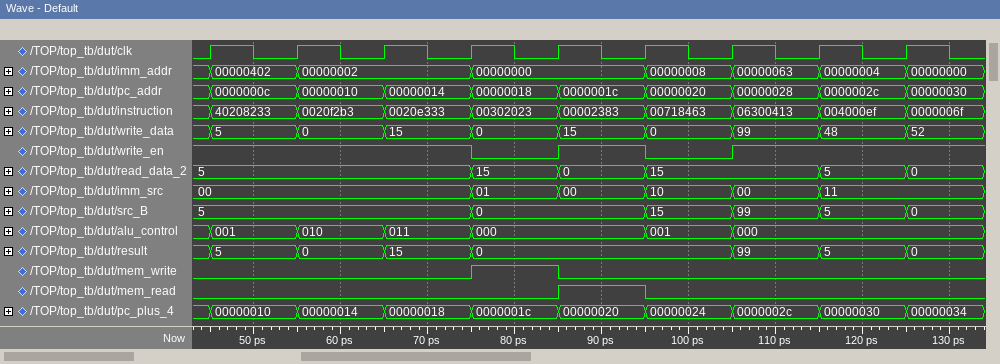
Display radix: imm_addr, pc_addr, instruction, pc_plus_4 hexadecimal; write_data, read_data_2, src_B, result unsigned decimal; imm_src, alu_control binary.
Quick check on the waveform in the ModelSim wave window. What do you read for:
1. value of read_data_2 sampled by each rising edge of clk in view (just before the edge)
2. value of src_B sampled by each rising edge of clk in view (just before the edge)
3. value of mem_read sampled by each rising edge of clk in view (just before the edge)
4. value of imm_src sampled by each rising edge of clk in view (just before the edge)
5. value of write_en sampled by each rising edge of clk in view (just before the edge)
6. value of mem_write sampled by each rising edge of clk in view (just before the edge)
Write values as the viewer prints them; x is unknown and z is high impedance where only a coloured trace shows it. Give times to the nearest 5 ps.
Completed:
5, 5, 5, 5, 15, 0, 15, 15, 5
5, 5, 5, 5, 0, 0, 15, 99, 5
0 0 0 0 0 1 0 0 0
00, 00, 00, 00, 01, 00, 10, 00, 11
1 1 1 1 0 1 0 1 1
0 0 0 0 1 0 0 0 0
